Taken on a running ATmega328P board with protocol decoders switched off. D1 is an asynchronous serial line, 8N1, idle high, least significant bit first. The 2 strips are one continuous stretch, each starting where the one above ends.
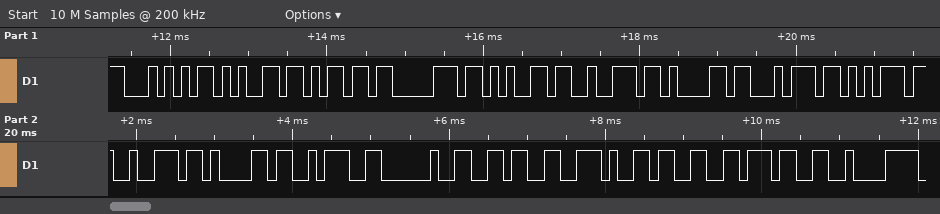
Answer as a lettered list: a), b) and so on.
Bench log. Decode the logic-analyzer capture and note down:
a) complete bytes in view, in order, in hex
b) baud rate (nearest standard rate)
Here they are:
a) 54 65 6D 70 65 72 61 74 75 72 61 3A 20 36 2E 33 37 C2
b) 9600 baud
